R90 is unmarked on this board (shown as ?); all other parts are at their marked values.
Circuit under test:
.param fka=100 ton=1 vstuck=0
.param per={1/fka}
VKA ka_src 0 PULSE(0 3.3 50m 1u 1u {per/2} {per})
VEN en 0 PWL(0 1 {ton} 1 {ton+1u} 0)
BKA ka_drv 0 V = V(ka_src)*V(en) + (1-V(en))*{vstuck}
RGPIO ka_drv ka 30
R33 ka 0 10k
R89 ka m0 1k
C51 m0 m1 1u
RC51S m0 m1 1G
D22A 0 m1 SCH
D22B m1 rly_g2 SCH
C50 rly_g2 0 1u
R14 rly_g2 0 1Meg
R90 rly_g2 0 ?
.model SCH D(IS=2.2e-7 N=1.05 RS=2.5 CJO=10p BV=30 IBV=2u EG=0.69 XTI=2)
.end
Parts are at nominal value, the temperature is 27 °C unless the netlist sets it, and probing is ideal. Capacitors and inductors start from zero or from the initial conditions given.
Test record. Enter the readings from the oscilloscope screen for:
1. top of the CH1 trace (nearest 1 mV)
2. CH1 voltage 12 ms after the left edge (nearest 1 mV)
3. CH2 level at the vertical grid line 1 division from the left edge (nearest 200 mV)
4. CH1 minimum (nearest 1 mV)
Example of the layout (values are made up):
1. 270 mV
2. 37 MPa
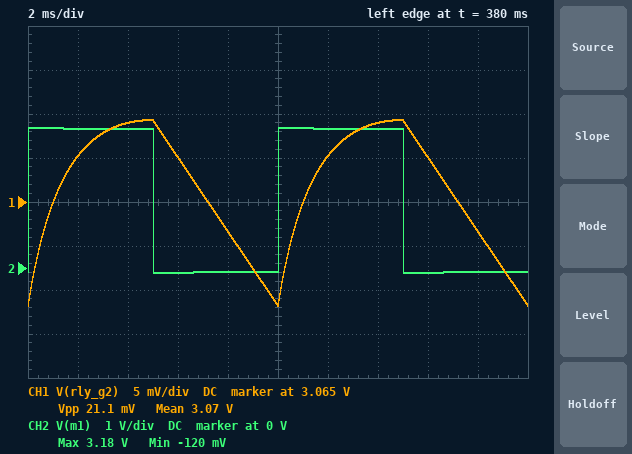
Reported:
1. 3.074 V
2. 3.070 V
3. 3.2 V
4. 3.053 V
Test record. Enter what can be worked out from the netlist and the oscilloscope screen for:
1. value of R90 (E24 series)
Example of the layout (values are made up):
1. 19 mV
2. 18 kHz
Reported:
1. 3.3 MΩ
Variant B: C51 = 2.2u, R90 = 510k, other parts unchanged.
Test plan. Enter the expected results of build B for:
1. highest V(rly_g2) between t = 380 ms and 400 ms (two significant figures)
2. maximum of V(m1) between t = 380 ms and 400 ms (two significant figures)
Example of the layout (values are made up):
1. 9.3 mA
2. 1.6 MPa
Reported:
1. 3.0 V
2. 3.1 V
